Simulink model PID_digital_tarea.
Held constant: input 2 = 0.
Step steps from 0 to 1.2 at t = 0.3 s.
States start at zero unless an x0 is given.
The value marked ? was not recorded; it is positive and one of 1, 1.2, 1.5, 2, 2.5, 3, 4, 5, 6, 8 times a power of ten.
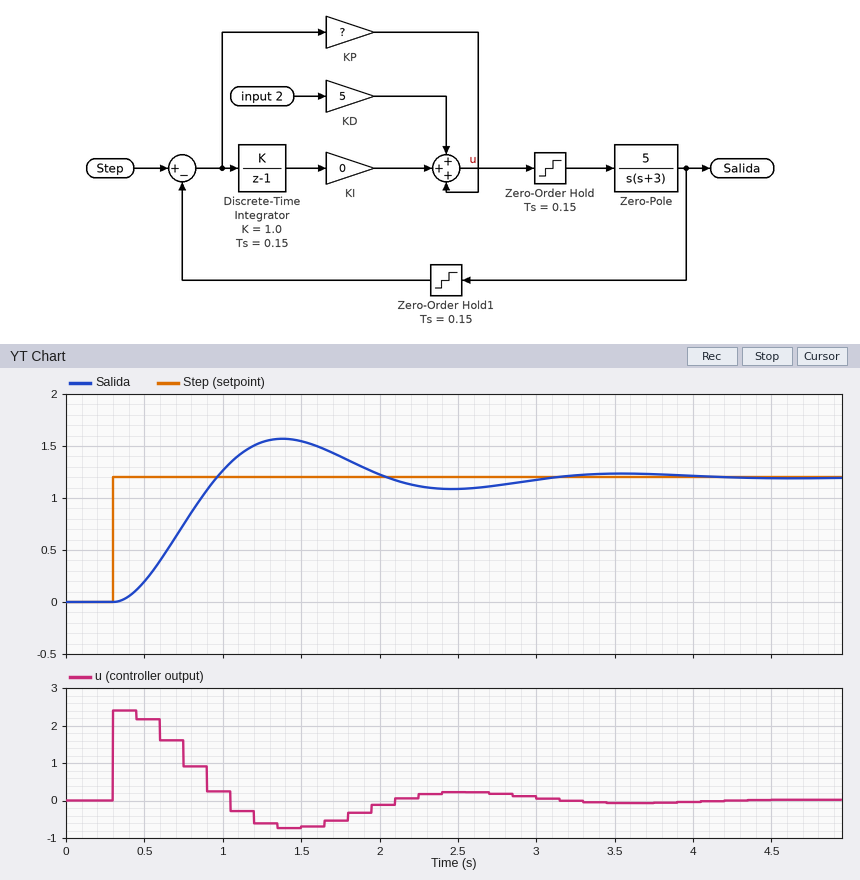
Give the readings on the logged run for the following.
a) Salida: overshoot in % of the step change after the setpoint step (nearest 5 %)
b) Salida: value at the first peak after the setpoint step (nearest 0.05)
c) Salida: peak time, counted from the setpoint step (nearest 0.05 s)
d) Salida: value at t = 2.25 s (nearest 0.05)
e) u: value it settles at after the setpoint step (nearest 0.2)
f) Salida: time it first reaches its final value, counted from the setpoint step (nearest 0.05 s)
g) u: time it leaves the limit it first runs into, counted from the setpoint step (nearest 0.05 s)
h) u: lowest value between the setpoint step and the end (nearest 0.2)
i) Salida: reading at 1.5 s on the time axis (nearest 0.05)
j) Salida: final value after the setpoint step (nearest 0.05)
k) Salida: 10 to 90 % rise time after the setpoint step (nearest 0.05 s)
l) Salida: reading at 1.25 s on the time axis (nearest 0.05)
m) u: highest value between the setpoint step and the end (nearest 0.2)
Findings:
30 %
1.55
1.10 s
1.10
0.0
0.65 s
0.15 s
-0.8
1.55
1.20
0.45 s
1.55
2.4
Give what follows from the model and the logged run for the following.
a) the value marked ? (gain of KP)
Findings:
2
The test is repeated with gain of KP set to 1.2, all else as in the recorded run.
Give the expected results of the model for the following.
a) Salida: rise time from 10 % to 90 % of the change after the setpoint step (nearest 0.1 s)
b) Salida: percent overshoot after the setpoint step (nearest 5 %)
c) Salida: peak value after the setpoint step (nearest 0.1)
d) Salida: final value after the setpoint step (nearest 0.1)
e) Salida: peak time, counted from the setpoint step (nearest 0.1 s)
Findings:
0.7 s
15 %
1.4
1.2
1.5 s
